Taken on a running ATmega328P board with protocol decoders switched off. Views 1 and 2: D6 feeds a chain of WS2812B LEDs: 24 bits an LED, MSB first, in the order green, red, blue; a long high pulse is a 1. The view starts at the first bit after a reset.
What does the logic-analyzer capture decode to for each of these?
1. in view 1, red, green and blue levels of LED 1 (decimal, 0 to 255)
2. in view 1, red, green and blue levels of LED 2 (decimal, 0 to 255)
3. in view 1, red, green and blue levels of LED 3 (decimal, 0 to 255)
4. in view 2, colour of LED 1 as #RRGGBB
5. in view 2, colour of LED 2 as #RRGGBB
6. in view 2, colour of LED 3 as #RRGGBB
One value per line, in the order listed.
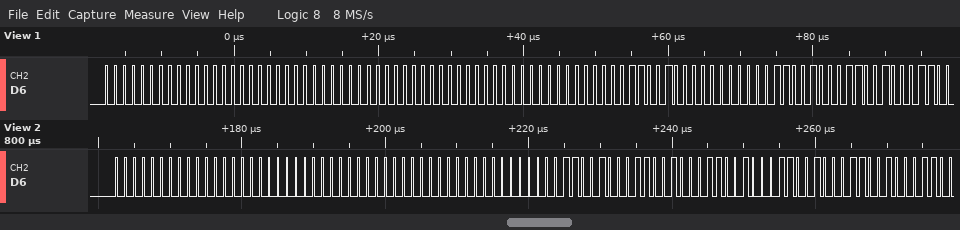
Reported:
0, 0, 0
0, 0, 0
50, 0, 0
#000000
#000000
#323232
